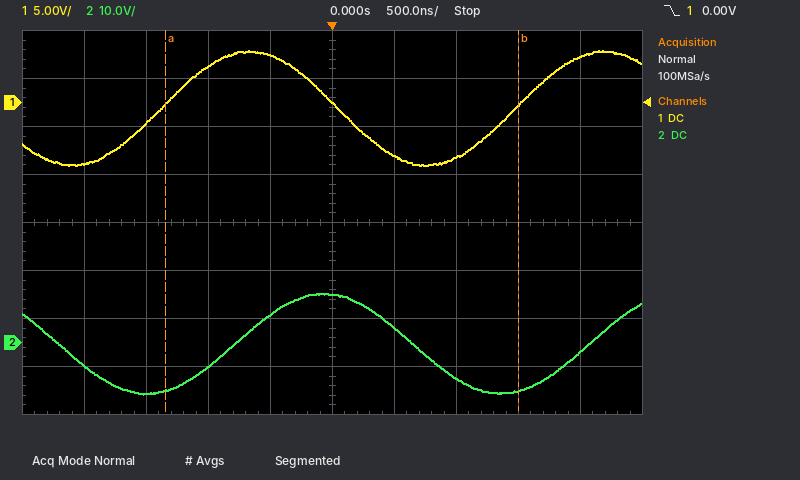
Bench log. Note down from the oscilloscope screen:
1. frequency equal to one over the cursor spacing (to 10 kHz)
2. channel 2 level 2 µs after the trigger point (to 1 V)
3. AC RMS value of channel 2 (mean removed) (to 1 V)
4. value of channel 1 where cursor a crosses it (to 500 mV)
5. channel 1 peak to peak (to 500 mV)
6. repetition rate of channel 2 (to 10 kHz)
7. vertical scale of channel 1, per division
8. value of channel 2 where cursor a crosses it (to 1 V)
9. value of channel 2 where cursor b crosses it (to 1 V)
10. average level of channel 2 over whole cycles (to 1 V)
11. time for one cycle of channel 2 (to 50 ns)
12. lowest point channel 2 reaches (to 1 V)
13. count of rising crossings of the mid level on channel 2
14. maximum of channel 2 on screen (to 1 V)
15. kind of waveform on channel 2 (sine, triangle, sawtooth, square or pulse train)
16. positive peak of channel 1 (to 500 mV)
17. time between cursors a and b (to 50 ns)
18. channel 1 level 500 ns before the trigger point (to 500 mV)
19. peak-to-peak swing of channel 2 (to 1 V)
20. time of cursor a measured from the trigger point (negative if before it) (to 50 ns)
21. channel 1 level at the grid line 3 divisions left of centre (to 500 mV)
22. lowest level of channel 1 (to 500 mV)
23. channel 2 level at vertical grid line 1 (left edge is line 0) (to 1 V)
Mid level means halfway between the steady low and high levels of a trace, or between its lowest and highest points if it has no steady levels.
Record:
350 kHz
-2 V
7 V
0.0 V
12.0 V
350 kHz
5 V
-10 V
-10 V
0 V
2.85 µs
-11 V
2
10 V
sine
5.5 V
2.85 µs
5.0 V
21 V
-1.35 µs
-2.0 V
-6.5 V
-5 V
